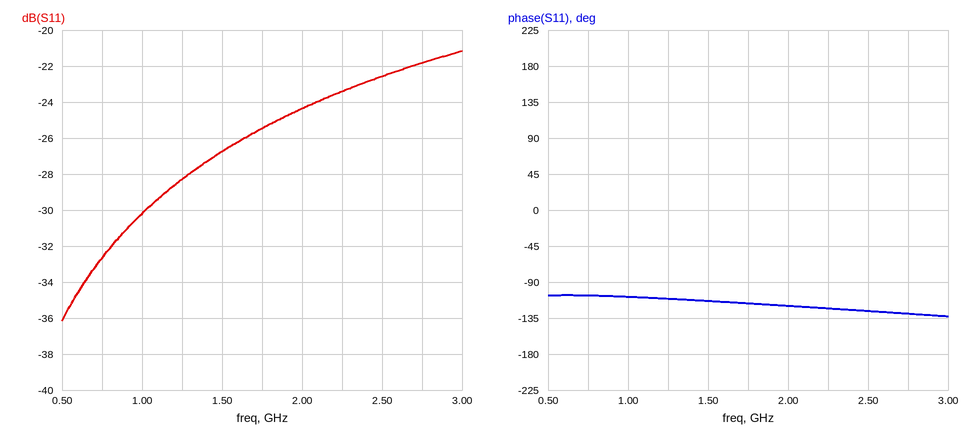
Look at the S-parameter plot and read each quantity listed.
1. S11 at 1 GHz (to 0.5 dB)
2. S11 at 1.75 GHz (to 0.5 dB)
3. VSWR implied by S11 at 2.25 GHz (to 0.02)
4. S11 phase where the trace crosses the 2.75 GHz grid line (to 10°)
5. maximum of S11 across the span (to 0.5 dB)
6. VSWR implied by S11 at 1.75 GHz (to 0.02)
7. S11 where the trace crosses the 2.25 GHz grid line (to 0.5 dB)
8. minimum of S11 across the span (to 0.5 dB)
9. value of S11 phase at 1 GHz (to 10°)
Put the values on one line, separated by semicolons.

-30.0 dB; -25.5 dB; 1.14; -130°; -21.0 dB; 1.12; -23.5 dB; -36.0 dB; -110°
